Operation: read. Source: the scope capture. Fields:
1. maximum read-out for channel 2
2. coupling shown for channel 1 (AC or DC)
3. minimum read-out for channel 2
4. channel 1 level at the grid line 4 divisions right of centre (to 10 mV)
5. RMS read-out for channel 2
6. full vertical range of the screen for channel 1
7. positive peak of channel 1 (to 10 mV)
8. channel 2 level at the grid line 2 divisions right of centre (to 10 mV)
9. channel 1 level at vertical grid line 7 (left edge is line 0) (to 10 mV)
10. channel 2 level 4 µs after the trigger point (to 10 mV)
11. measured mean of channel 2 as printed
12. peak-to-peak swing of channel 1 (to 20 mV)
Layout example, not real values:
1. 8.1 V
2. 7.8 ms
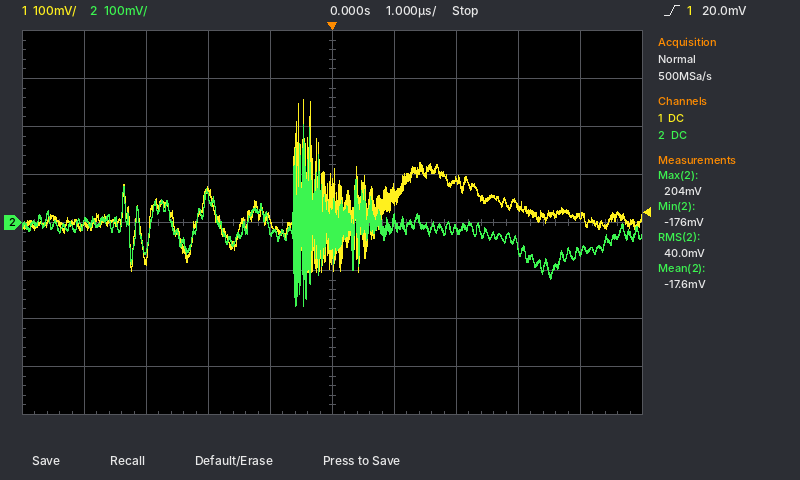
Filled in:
1. 204 mV
2. DC
3. -176 mV
4. 10 mV
5. 40.0 mV
6. 800 mV
7. 260 mV
8. -10 mV
9. 90 mV
10. -60 mV
11. -17.6 mV
12. 360 mV
